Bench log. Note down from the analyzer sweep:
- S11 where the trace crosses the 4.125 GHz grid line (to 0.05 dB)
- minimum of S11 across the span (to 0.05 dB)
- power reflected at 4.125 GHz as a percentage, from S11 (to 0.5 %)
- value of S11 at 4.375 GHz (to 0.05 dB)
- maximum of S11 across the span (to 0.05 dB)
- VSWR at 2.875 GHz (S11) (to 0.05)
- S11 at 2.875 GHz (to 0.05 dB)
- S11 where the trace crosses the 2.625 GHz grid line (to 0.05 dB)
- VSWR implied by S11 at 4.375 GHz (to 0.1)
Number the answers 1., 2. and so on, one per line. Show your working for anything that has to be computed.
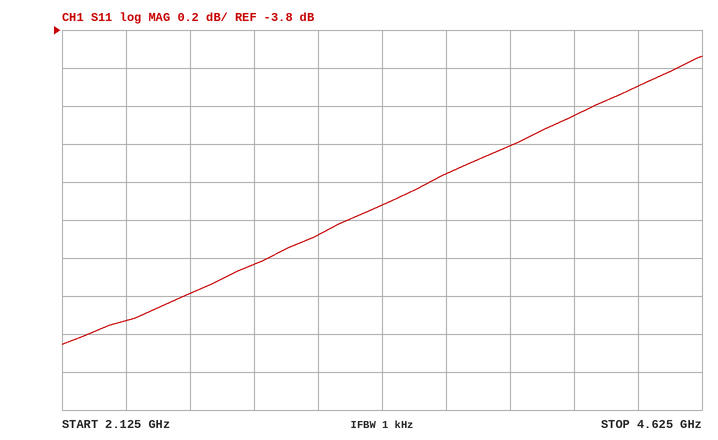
1. -4.25 dB
2. -5.45 dB
3. 10^(-4.25/10) ≈ 37.6 %, so 37.5 % to the nearest 0.5 %
4. -4.10 dB
5. -3.95 dB
6. |Γ| = 10^(-5.05/20) = 0.5591; VSWR = (1 + 0.5591)/(1 − 0.5591) ≈ 3.54, so 3.55 to the nearest 0.05
7. -5.05 dB
8. -5.20 dB
9. |Γ| = 10^(-4.1/20) = 0.6237; VSWR = (1 + 0.6237)/(1 − 0.6237) ≈ 4.3
